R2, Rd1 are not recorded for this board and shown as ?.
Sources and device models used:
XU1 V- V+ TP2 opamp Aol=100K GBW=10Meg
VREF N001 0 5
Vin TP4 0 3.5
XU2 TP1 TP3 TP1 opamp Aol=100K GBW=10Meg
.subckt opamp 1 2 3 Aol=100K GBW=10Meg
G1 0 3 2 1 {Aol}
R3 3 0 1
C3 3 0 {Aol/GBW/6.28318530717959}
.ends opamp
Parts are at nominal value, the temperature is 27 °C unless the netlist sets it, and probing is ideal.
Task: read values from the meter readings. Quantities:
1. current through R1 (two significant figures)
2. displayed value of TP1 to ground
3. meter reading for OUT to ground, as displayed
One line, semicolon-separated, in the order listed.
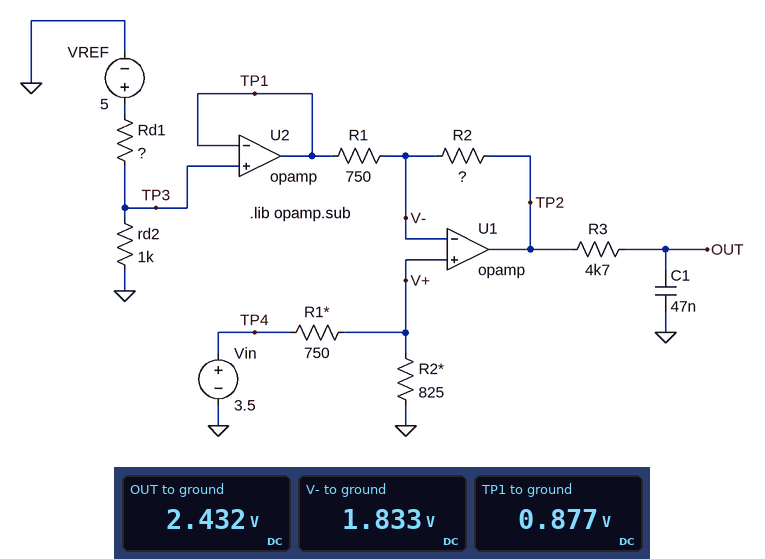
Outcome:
1.3 mA; 0.877 V; 2.432 V
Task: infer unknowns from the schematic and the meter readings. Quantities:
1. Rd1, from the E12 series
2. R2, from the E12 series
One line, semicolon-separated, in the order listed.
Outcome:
4.7 kΩ; 470 Ω
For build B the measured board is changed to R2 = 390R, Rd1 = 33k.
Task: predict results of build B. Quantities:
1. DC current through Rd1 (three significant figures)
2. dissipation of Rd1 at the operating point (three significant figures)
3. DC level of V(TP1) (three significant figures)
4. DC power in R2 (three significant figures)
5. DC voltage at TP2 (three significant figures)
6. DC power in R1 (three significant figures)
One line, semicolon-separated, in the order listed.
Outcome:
147 µA; 714 µW; 147 mV; 1.97 mW; 2.71 V; 3.79 mW
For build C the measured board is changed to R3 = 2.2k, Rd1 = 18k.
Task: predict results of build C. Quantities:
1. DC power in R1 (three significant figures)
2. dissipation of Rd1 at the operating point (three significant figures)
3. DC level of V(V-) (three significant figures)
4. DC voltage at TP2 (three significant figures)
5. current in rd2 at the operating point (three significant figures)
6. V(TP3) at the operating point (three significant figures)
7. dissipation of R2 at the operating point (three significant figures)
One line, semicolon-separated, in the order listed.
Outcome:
3.29 mW; 1.25 mW; 1.83 V; 2.82 V; 263 µA; 263 mV; 2.06 mW
